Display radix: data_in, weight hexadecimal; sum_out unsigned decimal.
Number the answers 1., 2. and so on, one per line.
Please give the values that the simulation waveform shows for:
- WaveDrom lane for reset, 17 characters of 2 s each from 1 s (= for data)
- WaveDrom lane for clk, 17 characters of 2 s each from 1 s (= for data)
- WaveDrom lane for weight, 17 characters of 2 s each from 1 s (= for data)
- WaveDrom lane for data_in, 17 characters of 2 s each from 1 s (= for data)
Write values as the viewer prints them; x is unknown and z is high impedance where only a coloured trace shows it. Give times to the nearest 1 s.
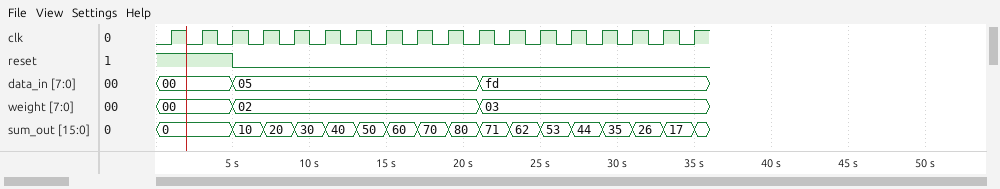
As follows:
1. {name: 'reset', wave: '1.0..............'}
2. {name: 'clk', wave: 'p................'}
3. {name: 'weight', wave: '=.=.......=......', data: '00 02 03'}
4. {name: 'data_in', wave: '=.=.......=......', data: '00 05 fd'}
